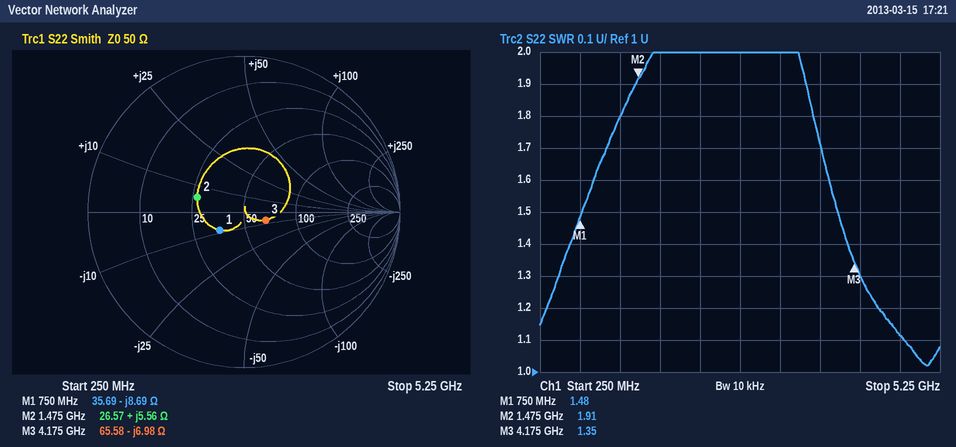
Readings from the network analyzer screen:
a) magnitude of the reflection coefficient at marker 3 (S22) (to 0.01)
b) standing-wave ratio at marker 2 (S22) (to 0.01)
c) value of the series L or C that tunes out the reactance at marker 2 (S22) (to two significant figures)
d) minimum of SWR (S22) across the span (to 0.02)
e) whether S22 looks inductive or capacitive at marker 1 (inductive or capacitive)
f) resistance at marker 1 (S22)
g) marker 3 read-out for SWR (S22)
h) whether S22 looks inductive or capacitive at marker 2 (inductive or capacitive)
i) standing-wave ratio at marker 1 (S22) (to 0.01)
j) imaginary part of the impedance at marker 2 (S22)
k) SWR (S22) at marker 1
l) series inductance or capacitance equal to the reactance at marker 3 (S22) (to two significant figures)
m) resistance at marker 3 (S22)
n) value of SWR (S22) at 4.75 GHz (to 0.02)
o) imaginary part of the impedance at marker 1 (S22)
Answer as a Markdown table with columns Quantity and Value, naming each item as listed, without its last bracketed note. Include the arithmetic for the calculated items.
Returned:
| Quantity | Value |
|---|---|
| magnitude of the reflection coefficient at marker 3 (S22) | 0.15 |
| standing-wave ratio at marker 2 (S22) | 1.91 |
| value of the series L or C that tunes out the reactance at marker 2 (S22) | C = 1/(2π × 1.475 GHz × 5.56 Ω) ≈ 19 pF |
| minimum of SWR (S22) across the span | 1.02 |
| whether S22 looks inductive or capacitive at marker 1 | capacitive |
| resistance at marker 1 | 35.69 Ω |
| marker 3 read-out for SWR | 1.35 |
| whether S22 looks inductive or capacitive at marker 2 | inductive |
| standing-wave ratio at marker 1 (S22) | 1.48 |
| imaginary part of the impedance at marker 2 | +5.56 Ω |
| SWR (S22) at marker 1 | 1.48 |
| series inductance or capacitance equal to the reactance at marker 3 (S22) | C = 1/(2π × 4.175 GHz × 6.98 Ω) ≈ 5.5 pF |
| resistance at marker 3 | 65.58 Ω |
| value of SWR (S22) at 4.75 GHz | 1.12 |
| imaginary part of the impedance at marker 1 | -8.69 Ω |
